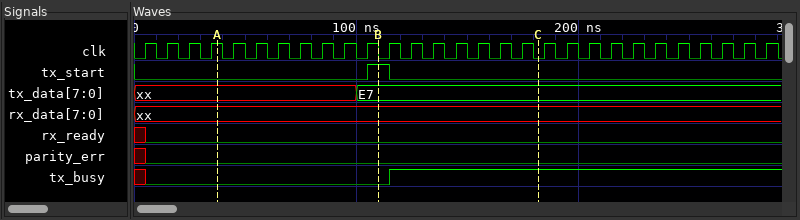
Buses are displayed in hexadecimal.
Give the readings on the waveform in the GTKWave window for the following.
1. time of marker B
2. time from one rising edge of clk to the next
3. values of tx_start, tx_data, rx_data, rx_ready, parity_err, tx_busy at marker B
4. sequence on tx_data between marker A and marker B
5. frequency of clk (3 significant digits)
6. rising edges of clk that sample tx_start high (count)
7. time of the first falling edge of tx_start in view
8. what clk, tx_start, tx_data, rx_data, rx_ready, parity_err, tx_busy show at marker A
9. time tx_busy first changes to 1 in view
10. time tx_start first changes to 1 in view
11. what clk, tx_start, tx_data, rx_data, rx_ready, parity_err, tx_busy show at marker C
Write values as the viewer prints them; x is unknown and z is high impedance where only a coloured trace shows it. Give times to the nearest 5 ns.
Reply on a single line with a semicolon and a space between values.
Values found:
110 ns; 10 ns; tx_start=1, tx_data=E7, rx_data=xx, rx_ready=0, parity_err=0, tx_busy=0; xx, E7; 100 MHz; 1; 115 ns; clk=1, tx_start=0, tx_data=xx, rx_data=xx, rx_ready=0, parity_err=0, tx_busy=0; 115 ns; 105 ns; clk=0, tx_start=0, tx_data=E7, rx_data=xx, rx_ready=0, parity_err=0, tx_busy=1
